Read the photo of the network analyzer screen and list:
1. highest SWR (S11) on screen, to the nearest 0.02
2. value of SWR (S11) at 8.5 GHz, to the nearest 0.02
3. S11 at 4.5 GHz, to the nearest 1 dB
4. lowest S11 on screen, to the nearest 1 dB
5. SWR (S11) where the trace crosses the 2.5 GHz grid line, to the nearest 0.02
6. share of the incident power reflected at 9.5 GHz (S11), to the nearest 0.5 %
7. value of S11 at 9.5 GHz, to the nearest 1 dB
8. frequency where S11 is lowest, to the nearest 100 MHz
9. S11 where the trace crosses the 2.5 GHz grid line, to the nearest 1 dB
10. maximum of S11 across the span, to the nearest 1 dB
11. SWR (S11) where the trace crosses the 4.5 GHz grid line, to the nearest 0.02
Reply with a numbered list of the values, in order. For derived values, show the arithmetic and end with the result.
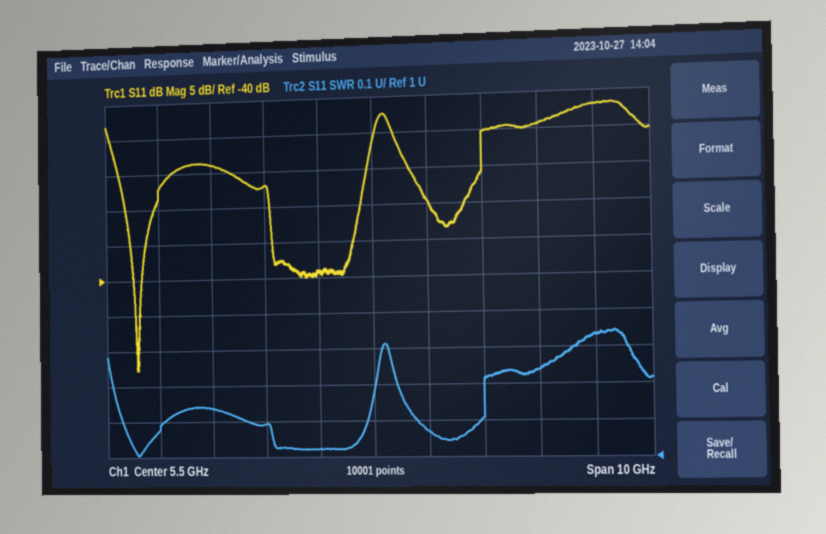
1. 1.34
2. 1.24
3. -39 dB
4. -53 dB
5. 1.14
6. 10^(-17/10) ≈ 2.0 %
7. -17 dB
8. 1.1 GHz
9. -24 dB
10. -17 dB
11. 1.02
